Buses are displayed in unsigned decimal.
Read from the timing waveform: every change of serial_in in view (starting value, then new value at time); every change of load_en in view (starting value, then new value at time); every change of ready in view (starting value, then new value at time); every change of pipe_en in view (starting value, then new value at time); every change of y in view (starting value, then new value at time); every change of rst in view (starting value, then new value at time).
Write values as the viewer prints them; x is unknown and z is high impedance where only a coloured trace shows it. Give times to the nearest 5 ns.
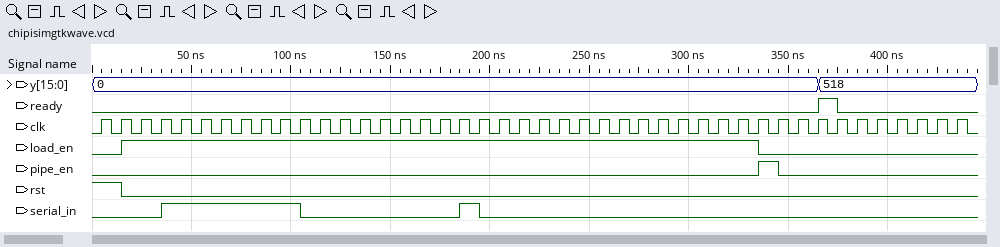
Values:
0, 1 at 35 ns, 0 at 105 ns, 1 at 185 ns, 0 at 195 ns
0, 1 at 15 ns, 0 at 335 ns
0, 1 at 365 ns, 0 at 375 ns
0, 1 at 335 ns, 0 at 345 ns
0, 518 at 365 ns
1, 0 at 15 ns
